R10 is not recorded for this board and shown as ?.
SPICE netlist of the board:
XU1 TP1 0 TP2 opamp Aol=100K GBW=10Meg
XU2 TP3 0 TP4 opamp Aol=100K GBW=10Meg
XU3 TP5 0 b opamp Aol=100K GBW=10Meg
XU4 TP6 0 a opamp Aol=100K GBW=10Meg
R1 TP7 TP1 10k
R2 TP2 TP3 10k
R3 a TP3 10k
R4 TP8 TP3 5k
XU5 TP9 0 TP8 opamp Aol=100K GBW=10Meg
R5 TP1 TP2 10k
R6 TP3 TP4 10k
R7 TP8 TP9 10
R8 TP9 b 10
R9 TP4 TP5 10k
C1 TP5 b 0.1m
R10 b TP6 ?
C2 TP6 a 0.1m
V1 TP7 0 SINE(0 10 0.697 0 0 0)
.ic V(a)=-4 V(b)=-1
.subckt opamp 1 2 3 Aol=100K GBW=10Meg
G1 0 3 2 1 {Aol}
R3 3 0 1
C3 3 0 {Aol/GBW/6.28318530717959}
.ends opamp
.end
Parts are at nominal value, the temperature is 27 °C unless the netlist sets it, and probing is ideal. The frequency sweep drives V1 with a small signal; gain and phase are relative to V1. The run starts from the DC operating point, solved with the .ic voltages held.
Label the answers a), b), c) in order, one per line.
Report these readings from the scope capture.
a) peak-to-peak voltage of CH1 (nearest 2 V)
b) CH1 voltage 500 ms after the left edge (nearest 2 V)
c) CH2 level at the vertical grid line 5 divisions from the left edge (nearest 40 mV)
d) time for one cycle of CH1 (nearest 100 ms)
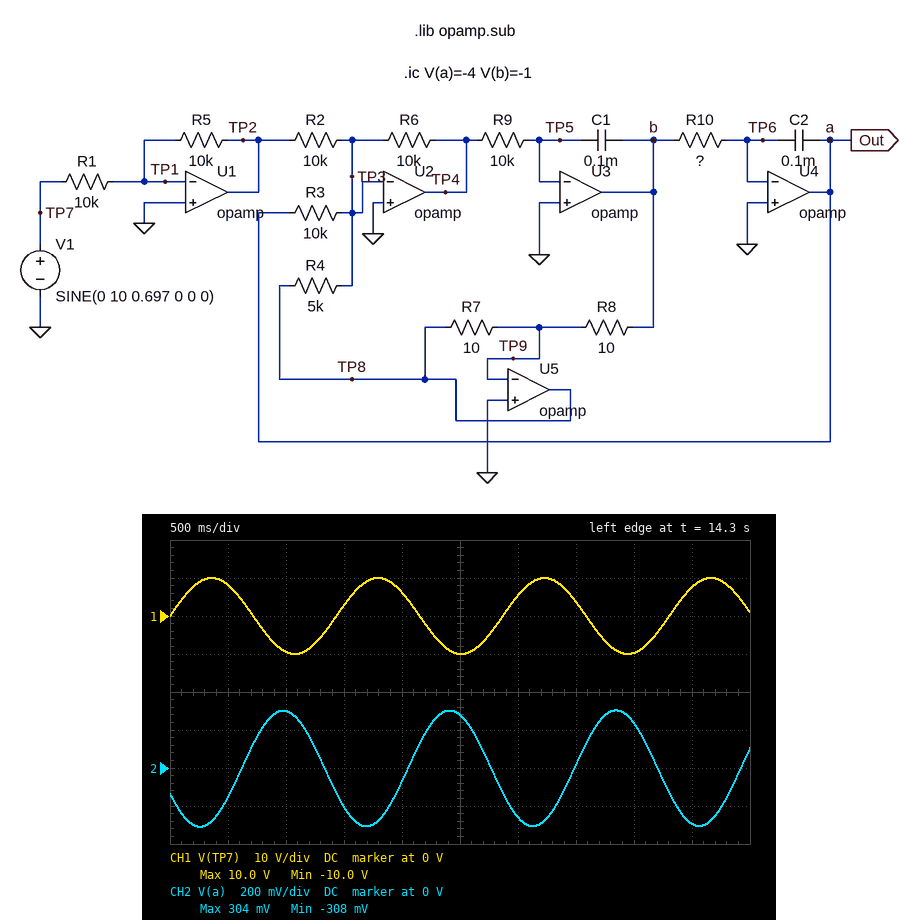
a) 20 V
b) 8 V
c) 280 mV
d) 1.4 s
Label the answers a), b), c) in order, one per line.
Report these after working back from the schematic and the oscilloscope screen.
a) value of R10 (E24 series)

a) 16 kΩ
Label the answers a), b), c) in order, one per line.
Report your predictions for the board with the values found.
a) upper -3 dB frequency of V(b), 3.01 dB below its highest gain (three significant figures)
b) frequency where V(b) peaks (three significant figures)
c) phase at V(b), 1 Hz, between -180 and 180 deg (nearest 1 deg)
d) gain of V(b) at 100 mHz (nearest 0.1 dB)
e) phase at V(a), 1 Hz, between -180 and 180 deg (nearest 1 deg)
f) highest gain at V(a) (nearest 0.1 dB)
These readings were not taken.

a) 362 mHz
b) 126 mHz
c) 108 deg
d) -6.2 dB
e) -162 deg
f) 0 dB
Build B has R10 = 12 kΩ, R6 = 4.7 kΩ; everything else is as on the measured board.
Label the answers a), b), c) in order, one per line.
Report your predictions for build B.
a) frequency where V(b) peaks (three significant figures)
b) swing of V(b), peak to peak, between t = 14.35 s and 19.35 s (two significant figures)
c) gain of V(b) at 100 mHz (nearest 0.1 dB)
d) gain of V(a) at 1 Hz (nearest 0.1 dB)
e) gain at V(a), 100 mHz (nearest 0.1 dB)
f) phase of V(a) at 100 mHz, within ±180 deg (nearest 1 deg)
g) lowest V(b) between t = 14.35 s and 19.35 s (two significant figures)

a) 99.6 mHz
b) 2.1 V
c) -6.0 dB
d) -40.1 dB
e) -3.6 dB
f) -90 deg
g) -1.1 V
